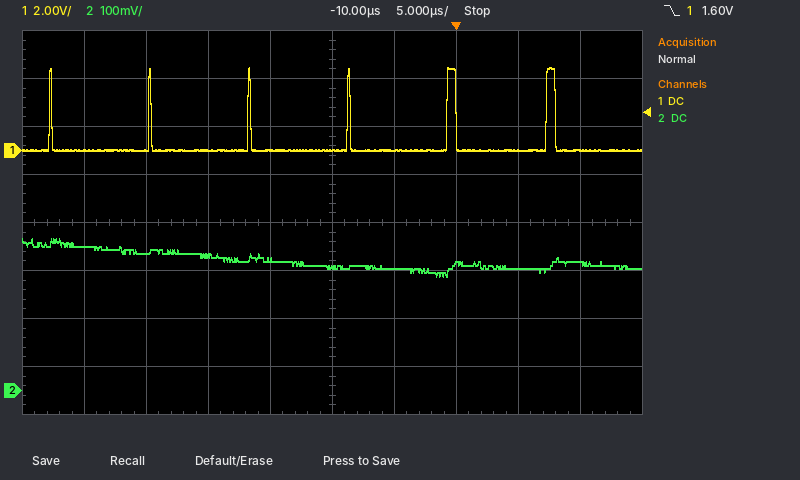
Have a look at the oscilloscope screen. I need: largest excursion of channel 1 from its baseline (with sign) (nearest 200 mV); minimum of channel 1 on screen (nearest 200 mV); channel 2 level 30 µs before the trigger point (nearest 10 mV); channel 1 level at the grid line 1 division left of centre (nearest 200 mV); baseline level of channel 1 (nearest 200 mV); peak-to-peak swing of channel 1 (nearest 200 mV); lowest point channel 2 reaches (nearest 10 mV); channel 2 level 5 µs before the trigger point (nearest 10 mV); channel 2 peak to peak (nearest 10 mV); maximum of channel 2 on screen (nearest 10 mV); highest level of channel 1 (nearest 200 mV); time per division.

+3.4 V
0.0 V
300 mV
0.0 V
0.0 V
3.4 V
240 mV
250 mV
80 mV
320 mV
3.4 V
5 µs
